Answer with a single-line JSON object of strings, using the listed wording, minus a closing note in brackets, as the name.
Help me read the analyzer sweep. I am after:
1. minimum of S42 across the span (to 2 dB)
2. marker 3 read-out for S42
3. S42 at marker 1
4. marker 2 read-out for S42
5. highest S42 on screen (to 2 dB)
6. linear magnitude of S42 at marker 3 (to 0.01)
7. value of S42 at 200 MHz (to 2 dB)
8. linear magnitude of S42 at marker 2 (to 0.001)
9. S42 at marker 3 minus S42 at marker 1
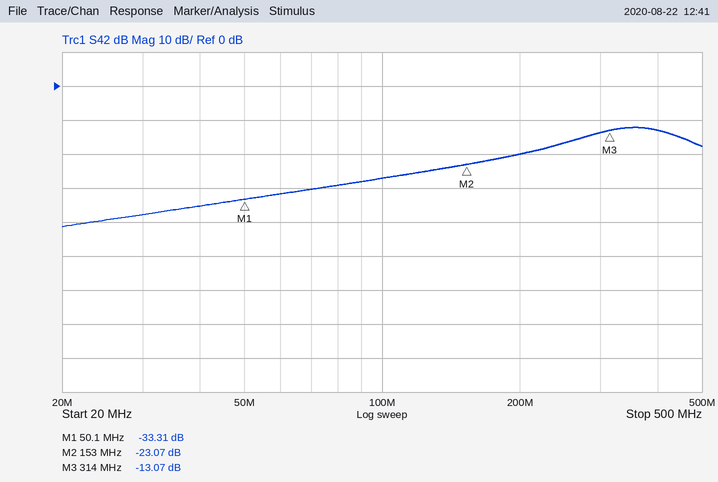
{"minimum of S42 across the span": "-42 dB", "marker 3 read-out for S42": "-13.07 dB", "S42 at marker 1": "-33.31 dB", "marker 2 read-out for S42": "-23.07 dB", "highest S42 on screen": "-12 dB", "linear magnitude of S42 at marker 3": "0.22", "value of S42 at 200 MHz": "-20 dB", "linear magnitude of S42 at marker 2": "0.070", "S42 at marker 3 minus S42 at marker 1": "20.24 dB"}
